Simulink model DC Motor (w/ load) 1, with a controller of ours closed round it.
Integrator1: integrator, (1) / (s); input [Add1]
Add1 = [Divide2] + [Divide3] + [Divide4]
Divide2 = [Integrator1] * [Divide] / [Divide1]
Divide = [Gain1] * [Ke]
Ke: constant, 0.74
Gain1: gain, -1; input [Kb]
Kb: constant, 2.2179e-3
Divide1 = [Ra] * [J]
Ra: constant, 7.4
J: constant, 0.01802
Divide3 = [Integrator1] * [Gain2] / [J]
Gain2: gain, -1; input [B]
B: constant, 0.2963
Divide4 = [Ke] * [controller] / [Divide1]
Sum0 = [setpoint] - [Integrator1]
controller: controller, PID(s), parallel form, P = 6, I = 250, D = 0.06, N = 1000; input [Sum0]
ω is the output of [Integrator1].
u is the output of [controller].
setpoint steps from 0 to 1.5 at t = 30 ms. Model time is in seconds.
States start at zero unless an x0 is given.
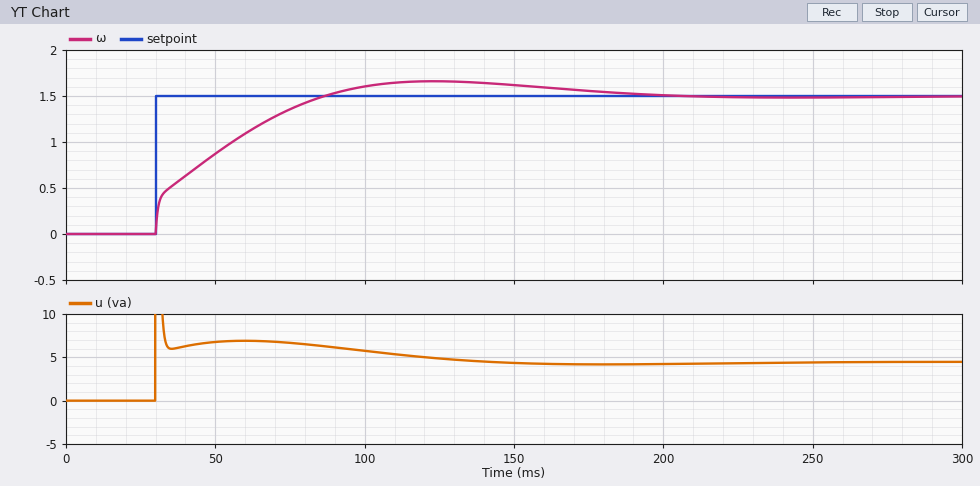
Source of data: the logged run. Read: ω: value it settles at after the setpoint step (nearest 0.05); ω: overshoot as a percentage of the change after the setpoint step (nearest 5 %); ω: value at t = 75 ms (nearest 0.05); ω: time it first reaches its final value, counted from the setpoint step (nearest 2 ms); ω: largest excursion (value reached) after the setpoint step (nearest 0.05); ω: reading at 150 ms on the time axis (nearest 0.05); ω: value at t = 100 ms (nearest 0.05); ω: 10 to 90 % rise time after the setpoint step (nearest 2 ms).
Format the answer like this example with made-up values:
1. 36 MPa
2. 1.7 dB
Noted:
1. 1.50
2. 10 %
3. 1.35
4. 56 ms
5. 1.65
6. 1.60
7. 1.60
8. 44 ms
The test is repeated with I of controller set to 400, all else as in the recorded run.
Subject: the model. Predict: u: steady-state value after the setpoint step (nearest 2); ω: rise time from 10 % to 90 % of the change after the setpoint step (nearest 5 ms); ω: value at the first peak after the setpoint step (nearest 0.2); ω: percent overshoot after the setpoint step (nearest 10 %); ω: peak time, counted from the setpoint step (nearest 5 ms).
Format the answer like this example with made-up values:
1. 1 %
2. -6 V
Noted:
1. 4
2. 35 ms
3. 1.8
4. 20 %
5. 70 ms
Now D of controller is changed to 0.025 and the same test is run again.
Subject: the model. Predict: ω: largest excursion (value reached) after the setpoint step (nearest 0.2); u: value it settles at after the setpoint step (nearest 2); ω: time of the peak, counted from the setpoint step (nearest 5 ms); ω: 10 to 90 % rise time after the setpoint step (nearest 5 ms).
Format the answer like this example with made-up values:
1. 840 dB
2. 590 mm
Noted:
1. 1.6
2. 4
3. 85 ms
4. 40 ms
